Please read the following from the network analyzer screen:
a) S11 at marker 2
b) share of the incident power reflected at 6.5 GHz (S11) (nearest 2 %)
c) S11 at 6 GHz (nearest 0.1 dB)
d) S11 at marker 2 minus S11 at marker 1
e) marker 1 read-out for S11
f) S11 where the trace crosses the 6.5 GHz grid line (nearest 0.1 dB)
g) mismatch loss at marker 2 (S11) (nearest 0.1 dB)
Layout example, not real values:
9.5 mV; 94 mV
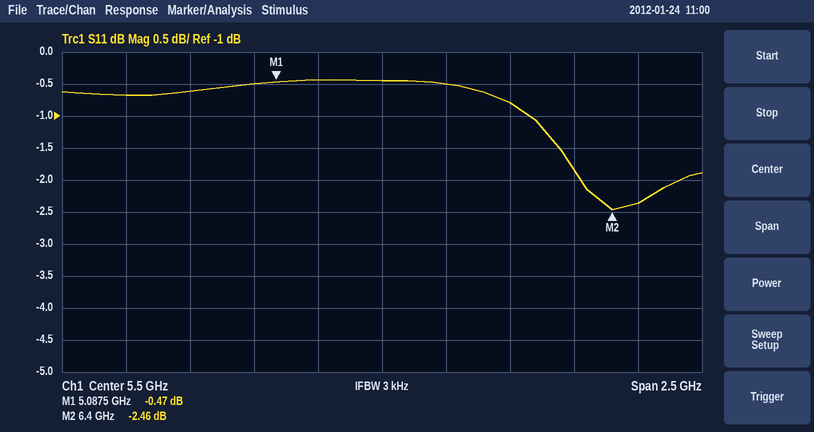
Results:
-2.46 dB; 58 %; -0.8 dB; -1.99 dB; -0.47 dB; -2.4 dB; 3.6 dB
